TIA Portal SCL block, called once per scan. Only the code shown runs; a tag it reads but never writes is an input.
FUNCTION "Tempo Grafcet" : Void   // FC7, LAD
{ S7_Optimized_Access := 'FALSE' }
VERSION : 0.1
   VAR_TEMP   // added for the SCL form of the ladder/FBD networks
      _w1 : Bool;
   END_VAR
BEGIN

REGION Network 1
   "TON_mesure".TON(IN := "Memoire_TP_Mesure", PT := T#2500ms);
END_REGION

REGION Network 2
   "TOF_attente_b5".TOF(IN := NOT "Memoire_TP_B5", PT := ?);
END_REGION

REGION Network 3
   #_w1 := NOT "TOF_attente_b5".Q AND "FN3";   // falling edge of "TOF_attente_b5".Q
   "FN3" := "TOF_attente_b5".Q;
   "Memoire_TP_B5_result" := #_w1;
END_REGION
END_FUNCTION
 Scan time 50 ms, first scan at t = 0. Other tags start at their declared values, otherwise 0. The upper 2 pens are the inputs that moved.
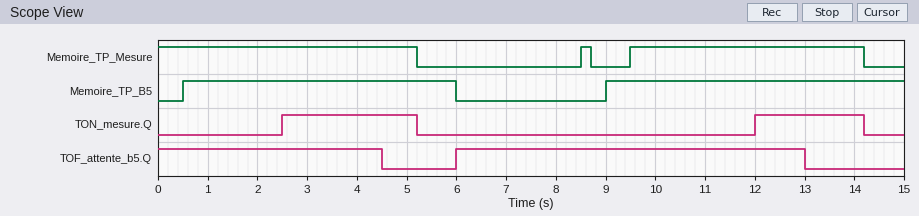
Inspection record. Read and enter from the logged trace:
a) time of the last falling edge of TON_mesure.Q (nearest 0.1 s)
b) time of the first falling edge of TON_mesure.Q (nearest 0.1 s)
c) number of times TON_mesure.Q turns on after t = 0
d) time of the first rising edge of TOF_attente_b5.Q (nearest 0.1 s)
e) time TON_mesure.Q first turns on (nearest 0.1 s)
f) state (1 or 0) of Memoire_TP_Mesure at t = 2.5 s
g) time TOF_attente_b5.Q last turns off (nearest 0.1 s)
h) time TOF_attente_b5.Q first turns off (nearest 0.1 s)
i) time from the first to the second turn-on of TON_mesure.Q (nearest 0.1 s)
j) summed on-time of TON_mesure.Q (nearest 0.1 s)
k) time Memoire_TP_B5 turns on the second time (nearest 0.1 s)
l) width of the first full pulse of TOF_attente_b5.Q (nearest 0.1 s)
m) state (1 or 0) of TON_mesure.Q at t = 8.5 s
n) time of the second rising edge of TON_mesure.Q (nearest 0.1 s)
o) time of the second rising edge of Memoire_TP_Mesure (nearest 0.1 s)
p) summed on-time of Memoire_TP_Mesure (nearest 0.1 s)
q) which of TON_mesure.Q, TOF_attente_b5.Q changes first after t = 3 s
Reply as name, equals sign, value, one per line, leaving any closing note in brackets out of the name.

time of the last falling edge of TON_mesure.Q = 14.2 s
time of the first falling edge of TON_mesure.Q = 5.2 s
number of times TON_mesure.Q turns on after t = 0 = 2
time of the first rising edge of TOF_attente_b5.Q = 6.0 s
time TON_mesure.Q first turns on = 2.5 s
state (1 or 0) of Memoire_TP_Mesure at t = 2.5 s = 1
time TOF_attente_b5.Q last turns off = 13.0 s
time TOF_attente_b5.Q first turns off = 4.5 s
time from the first to the second turn-on of TON_mesure.Q = 9.5 s
summed on-time of TON_mesure.Q = 4.9 s
time Memoire_TP_B5 turns on the second time = 9.0 s
width of the first full pulse of TOF_attente_b5.Q = 7.0 s
state (1 or 0) of TON_mesure.Q at t = 8.5 s = 0
time of the second rising edge of TON_mesure.Q = 12.0 s
time of the second rising edge of Memoire_TP_Mesure = 9.5 s
summed on-time of Memoire_TP_Mesure = 10.1 s
which of TON_mesure.Q, TOF_attente_b5.Q changes first after t = 3 s = TOF_attente_b5.Q
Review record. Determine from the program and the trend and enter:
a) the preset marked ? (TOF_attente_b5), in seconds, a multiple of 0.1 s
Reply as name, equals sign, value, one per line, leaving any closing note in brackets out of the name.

the preset marked ? (TOF_attente_b5), in seconds, a multiple of 0.1 s = 4.0 s
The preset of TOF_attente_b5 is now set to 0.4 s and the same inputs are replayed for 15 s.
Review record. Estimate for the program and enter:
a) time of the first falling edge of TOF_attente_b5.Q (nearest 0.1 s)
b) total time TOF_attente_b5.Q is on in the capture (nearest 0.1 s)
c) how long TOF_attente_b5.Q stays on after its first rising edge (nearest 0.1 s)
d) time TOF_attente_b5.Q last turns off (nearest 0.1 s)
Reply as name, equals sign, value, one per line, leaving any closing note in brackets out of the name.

time of the first falling edge of TOF_attente_b5.Q = 0.9 s
total time TOF_attente_b5.Q is on in the capture = 4.3 s
how long TOF_attente_b5.Q stays on after its first rising edge = 3.4 s
time TOF_attente_b5.Q last turns off = 9.4 s
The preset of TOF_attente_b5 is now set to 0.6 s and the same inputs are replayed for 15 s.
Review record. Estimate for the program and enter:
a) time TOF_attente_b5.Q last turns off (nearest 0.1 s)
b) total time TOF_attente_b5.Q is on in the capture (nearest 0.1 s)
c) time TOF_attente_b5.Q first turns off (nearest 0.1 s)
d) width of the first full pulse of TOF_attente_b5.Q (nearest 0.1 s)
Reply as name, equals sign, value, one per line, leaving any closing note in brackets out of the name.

time TOF_attente_b5.Q last turns off = 9.6 s
total time TOF_attente_b5.Q is on in the capture = 4.7 s
time TOF_attente_b5.Q first turns off = 1.1 s
width of the first full pulse of TOF_attente_b5.Q = 3.6 s
